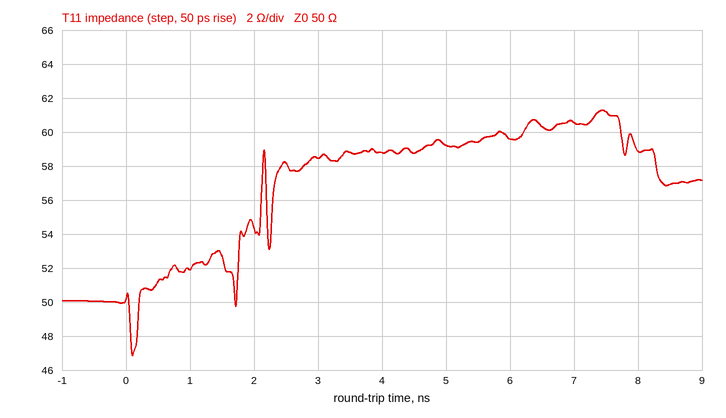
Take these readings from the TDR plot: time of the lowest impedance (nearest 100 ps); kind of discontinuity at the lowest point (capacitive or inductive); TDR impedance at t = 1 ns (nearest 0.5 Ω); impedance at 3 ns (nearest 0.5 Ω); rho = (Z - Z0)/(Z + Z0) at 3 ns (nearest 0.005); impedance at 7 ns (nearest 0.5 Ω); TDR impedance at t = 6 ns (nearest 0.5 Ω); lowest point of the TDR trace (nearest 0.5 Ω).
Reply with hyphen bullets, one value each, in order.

- 100 ps
- capacitive
- 52.0 Ω
- 58.5 Ω
- +0.080
- 60.5 Ω
- 59.5 Ω
- 47.0 Ω
